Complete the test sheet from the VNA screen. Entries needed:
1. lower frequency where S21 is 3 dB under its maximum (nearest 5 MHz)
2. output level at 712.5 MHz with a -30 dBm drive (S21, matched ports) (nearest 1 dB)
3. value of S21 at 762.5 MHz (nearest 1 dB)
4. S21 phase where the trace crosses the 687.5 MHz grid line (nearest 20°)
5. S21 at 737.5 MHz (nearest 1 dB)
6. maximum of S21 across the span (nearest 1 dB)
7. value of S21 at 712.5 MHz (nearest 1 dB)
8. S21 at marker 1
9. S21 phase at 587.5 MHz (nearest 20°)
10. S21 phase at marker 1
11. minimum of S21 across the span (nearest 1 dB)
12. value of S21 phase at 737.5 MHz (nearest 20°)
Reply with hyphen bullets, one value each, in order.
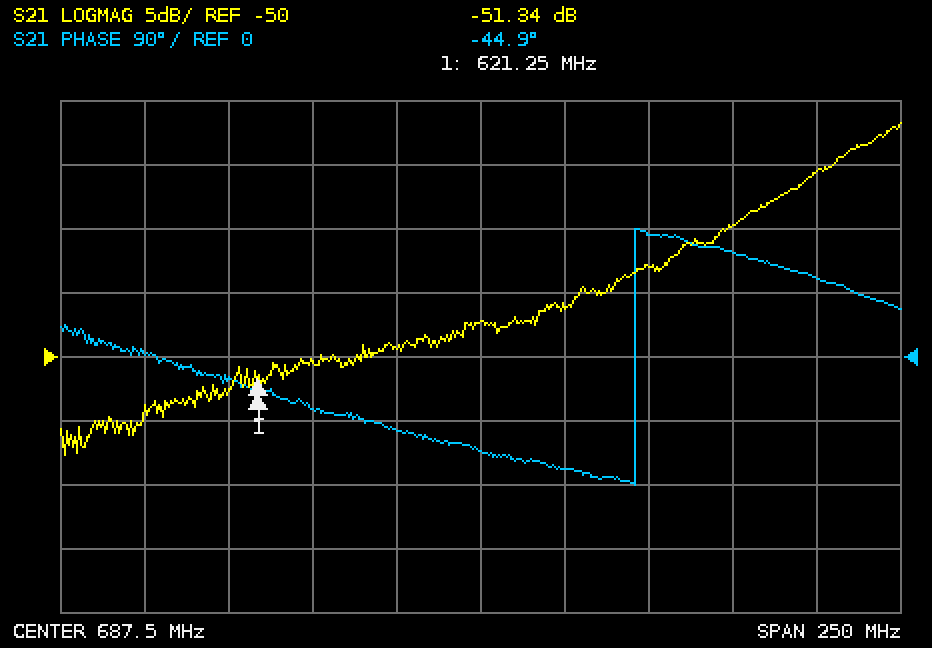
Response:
- 795 MHz
- -76 dBm
- -40 dB
- -140°
- -43 dB
- -32 dB
- -46 dB
- -51.34 dB
- 0°
- -44.9°
- -58 dB
- 180°
